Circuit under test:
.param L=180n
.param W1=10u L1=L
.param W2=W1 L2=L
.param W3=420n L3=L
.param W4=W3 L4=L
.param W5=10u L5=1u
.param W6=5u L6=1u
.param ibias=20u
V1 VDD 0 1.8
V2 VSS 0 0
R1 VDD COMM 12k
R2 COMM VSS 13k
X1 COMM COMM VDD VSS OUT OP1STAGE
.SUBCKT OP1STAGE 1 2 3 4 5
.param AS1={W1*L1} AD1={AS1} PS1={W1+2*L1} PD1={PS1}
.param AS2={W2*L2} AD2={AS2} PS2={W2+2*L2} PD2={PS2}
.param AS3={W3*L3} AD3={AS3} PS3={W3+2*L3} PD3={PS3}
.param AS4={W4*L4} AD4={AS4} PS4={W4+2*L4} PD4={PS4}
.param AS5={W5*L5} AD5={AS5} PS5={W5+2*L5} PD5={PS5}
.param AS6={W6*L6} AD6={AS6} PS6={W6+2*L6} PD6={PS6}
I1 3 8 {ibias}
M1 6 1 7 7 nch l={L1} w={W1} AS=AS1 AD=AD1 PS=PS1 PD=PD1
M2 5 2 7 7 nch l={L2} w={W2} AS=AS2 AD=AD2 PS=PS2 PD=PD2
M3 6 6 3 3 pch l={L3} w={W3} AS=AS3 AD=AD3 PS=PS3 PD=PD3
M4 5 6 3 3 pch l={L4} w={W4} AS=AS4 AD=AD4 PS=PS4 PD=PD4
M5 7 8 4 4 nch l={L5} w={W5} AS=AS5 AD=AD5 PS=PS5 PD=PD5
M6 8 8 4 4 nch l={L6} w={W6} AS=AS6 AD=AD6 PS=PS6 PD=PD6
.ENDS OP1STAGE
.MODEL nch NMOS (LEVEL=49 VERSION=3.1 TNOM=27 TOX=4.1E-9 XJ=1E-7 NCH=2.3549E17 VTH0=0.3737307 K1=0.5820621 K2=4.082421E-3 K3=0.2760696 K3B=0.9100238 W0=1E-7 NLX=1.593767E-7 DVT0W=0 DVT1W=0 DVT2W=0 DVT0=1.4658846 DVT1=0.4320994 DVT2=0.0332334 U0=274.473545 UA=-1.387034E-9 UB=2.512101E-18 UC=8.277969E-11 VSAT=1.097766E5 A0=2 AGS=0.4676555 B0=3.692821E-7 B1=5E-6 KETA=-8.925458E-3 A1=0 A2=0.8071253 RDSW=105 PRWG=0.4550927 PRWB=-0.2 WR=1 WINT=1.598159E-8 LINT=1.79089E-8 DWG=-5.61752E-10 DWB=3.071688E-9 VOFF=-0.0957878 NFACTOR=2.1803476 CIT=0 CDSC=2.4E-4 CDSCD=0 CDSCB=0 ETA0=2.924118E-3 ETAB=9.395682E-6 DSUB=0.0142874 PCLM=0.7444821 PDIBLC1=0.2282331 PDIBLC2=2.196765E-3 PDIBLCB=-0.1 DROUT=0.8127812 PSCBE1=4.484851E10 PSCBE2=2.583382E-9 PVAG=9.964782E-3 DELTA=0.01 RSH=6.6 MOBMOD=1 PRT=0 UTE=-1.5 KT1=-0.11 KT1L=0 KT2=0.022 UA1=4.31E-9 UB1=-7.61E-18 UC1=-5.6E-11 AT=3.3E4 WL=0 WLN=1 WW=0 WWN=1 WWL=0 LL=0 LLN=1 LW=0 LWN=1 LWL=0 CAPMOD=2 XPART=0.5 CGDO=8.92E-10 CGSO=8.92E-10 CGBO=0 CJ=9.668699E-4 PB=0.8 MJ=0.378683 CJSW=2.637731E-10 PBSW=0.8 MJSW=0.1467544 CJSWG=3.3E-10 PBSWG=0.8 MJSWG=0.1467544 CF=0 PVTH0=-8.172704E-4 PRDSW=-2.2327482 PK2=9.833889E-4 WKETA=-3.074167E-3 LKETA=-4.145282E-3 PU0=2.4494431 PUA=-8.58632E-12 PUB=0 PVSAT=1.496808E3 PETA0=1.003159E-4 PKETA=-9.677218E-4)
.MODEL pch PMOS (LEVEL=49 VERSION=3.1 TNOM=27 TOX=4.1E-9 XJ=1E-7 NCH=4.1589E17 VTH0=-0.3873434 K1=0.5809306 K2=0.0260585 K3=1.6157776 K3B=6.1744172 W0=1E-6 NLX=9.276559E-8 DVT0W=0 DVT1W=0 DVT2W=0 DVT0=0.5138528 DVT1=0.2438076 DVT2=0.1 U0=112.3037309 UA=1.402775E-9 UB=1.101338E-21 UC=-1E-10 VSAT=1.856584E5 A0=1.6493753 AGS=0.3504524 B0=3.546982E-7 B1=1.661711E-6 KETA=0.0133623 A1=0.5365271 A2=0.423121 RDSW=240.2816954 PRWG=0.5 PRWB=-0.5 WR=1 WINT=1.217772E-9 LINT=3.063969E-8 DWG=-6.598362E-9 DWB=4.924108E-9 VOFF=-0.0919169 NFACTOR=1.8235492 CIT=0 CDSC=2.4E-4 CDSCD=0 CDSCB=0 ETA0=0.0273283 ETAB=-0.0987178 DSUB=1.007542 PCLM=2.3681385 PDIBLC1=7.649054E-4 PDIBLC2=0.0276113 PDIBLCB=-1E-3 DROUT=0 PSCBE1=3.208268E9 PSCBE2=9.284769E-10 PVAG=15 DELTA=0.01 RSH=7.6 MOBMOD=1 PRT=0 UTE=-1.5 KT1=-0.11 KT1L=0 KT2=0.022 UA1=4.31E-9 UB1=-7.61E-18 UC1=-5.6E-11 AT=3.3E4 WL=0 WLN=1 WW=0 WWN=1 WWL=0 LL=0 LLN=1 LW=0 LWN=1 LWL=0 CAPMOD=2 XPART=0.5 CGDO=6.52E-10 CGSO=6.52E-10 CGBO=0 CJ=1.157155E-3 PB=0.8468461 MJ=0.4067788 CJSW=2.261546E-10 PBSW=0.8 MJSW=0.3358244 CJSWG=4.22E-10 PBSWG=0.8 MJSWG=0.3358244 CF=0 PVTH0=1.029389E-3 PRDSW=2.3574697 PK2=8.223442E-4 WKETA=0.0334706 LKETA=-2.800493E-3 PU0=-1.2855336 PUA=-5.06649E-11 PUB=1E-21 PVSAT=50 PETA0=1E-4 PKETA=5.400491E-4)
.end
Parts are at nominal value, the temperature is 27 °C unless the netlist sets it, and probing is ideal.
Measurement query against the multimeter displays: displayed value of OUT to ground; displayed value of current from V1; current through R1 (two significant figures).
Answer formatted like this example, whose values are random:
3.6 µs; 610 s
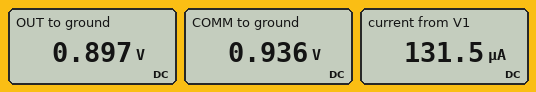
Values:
0.897 V; 131.5 µA; 72 µA
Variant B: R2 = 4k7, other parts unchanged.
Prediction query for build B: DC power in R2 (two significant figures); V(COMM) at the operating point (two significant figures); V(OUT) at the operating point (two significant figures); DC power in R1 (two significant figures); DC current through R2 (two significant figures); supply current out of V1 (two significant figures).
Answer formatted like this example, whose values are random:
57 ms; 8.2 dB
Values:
55 µW; 510 mV; 1.0 V; 140 µW; 110 µA; 150 µA
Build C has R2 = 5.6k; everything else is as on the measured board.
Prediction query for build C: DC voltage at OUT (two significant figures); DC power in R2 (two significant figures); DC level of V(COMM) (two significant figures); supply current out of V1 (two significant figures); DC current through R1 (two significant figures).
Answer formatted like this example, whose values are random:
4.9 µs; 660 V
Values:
950 mV; 59 µW; 570 mV; 150 µA; 100 µA
